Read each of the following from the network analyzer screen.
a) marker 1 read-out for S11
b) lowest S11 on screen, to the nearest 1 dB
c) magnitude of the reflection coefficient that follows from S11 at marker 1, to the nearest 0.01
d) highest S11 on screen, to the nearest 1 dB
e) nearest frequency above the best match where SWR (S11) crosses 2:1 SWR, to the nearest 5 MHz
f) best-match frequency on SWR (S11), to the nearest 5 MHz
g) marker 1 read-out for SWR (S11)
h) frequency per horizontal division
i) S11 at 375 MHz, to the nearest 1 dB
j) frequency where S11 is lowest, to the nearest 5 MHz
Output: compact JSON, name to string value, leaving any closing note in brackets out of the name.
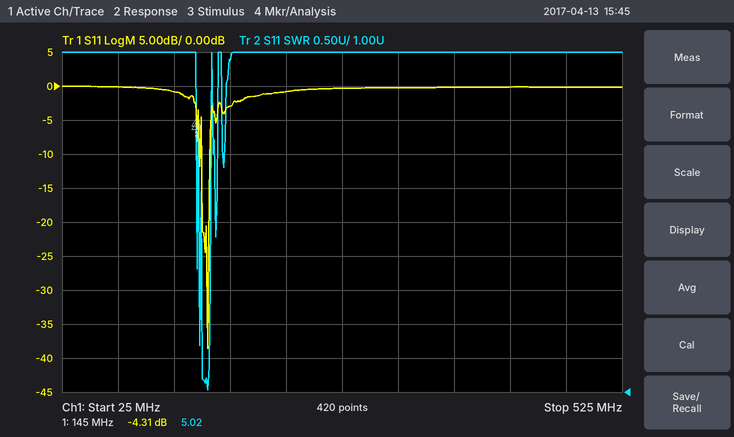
{"marker 1 read-out for S11": "-4.31 dB", "lowest S11 on screen, to the nearest 1 dB": "-39 dB", "magnitude of the reflection coefficient that follows from S11 at marker 1, to the nearest 0.01": "0.61", "highest S11 on screen, to the nearest 1 dB": "0 dB", "nearest frequency above the best match where SWR (S11) crosses 2:1 SWR, to the nearest 5 MHz": "155 MHz", "best-match frequency on SWR (S11), to the nearest 5 MHz": "155 MHz", "marker 1 read-out for SWR": "5.02", "frequency per horizontal division": "50 MHz", "S11 at 375 MHz, to the nearest 1 dB": "0 dB", "frequency where S11 is lowest, to the nearest 5 MHz": "155 MHz"}
